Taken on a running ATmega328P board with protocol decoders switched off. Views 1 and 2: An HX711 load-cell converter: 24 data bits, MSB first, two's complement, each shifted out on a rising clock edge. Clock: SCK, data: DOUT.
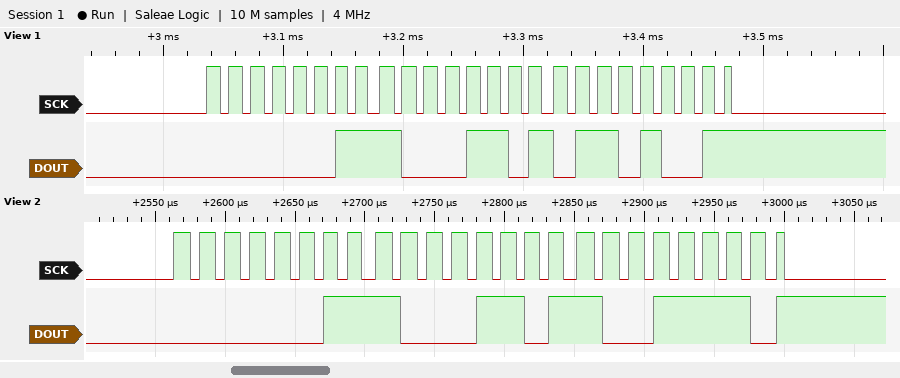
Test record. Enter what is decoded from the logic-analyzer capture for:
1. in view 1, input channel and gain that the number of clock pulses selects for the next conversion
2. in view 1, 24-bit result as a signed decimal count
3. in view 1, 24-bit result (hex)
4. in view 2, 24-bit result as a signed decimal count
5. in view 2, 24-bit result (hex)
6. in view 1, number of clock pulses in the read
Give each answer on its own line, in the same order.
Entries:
channel A, gain 128
232809
0x038D69
232862
0x038D9E
25
